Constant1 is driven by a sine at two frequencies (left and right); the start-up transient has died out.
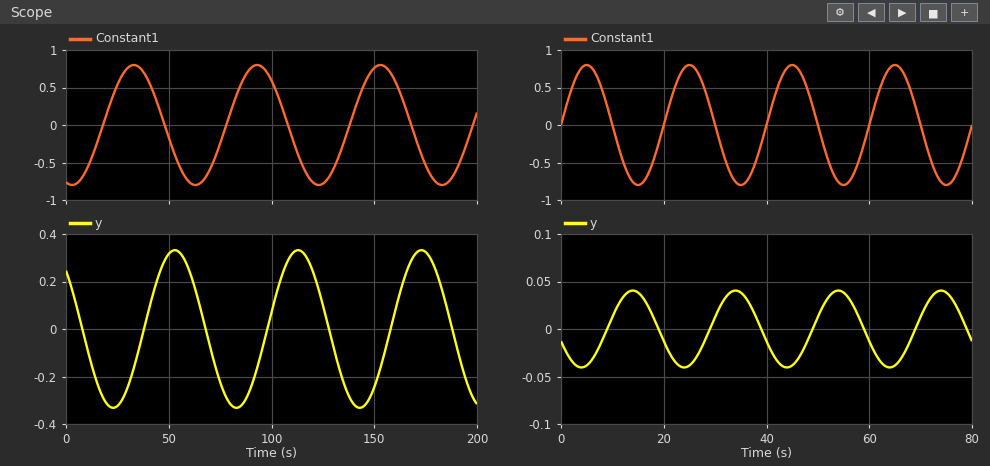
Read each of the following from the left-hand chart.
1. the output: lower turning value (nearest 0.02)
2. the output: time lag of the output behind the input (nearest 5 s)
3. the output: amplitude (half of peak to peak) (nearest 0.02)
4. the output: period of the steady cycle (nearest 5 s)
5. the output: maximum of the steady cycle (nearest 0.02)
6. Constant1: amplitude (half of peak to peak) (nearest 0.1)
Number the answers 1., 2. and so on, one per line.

1. -0.34
2. 20 s
3. 0.34
4. 60 s
5. 0.34
6. 0.8
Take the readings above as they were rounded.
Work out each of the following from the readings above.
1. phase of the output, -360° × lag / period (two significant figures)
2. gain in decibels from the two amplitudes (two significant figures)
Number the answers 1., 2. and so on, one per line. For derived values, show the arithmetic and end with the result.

1. -360 × 20 / 60 = -120°
2. 20 log10(0.34 / 0.8) = -7.4 dB
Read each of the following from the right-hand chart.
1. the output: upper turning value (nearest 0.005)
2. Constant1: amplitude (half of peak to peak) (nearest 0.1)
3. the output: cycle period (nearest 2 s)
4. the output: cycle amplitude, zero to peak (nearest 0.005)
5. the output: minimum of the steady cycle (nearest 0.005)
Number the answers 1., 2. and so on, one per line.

1. 0.040
2. 0.8
3. 20 s
4. 0.040
5. -0.040
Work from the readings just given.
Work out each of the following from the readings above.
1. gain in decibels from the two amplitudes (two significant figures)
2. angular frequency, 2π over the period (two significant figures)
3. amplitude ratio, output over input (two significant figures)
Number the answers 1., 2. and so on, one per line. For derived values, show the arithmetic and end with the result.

1. 20 log10(0.04 / 0.8) = -26 dB
2. 2π / 20 = 0.31 rad/s
3. 0.04 / 0.8 = 0.050
